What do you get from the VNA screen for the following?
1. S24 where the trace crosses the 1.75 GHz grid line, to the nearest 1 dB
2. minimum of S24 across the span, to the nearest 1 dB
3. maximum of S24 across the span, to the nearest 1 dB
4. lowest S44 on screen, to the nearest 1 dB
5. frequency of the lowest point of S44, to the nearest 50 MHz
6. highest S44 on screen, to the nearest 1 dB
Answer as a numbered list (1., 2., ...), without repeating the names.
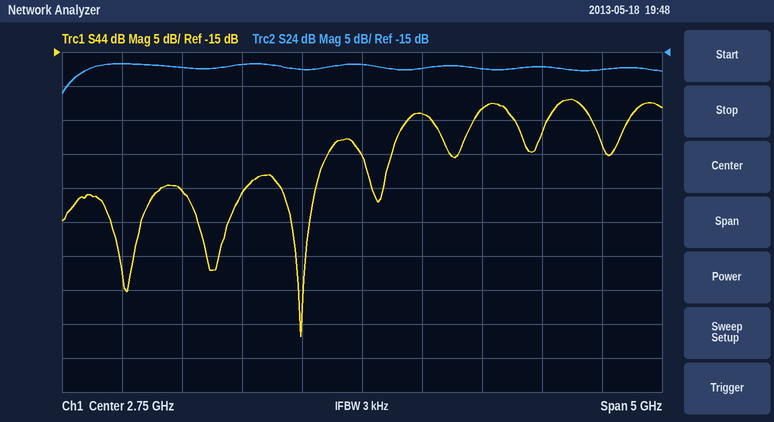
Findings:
1. -17 dB
2. -21 dB
3. -17 dB
4. -57 dB
5. 2.25 GHz
6. -22 dB
